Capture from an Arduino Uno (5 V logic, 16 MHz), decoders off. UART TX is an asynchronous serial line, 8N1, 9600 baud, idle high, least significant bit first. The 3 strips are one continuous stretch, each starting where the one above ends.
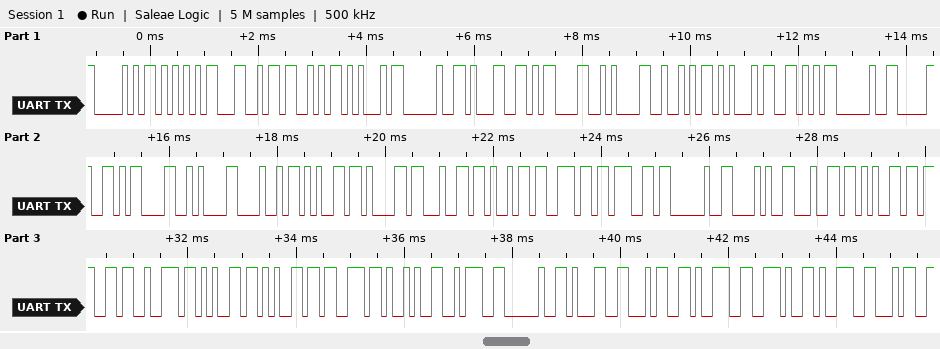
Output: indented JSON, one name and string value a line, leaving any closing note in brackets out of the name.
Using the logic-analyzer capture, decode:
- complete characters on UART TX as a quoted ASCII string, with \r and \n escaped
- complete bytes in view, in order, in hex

{
  "complete characters on UART TX as a quoted ASCII string, with \\r and \\n escaped": "\"PULSE 1\\r\\nREV 0\\r\\nHeading (degrees): 149.94\"",
  "complete bytes in view, in order, in hex": "0x50 0x55 0x4C 0x53 0x45 0x20 0x31 0x0D 0x0A 0x52 0x45 0x56 0x20 0x30 0x0D 0x0A 0x48 0x65 0x61 0x64 0x69 0x6E 0x67 0x20 0x28 0x64 0x65 0x67 0x72 0x65 0x65 0x73 0x29 0x3A 0x20 0x31 0x34 0x39 0x2E 0x39 0x34"
}
